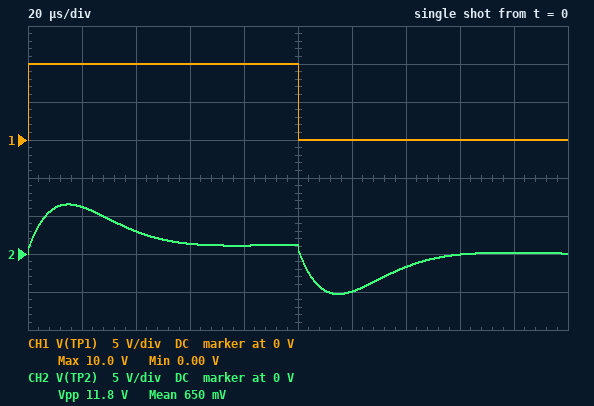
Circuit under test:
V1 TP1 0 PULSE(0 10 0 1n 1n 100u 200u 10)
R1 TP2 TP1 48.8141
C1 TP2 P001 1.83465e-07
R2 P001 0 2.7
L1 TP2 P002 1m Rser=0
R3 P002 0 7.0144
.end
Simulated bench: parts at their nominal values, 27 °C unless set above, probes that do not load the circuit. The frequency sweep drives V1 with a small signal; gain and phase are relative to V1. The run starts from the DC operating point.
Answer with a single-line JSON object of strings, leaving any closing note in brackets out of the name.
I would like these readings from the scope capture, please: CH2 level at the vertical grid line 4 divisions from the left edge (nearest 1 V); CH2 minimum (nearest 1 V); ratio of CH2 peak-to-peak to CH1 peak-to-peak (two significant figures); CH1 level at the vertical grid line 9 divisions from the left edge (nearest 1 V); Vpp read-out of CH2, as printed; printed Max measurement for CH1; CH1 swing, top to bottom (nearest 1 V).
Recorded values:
{"CH2 level at the vertical grid line 4 divisions from the left edge": "1 V", "CH2 minimum": "-5 V", "ratio of CH2 peak-to-peak to CH1 peak-to-peak": "1.2", "CH1 level at the vertical grid line 9 divisions from the left edge": "0 V", "Vpp read-out of CH2, as printed": "11.8 V", "printed Max measurement for CH1": "10.0 V", "CH1 swing, top to bottom": "10 V"}
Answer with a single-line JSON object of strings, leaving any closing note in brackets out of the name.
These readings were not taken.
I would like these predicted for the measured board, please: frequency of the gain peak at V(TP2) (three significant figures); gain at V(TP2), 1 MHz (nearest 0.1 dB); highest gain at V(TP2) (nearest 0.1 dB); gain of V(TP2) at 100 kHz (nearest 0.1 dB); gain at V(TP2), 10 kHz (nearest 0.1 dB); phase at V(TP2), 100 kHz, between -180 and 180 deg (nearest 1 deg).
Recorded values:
{"frequency of the gain peak at V(TP2)": "12.2 kHz", "gain at V(TP2), 1 MHz": "-25.2 dB", "highest gain at V(TP2)": "-0.7 dB", "gain of V(TP2) at 100 kHz": "-15.1 dB", "gain at V(TP2), 10 kHz": "-1.0 dB", "phase at V(TP2), 100 kHz, between -180 and 180 deg": "-63 deg"}
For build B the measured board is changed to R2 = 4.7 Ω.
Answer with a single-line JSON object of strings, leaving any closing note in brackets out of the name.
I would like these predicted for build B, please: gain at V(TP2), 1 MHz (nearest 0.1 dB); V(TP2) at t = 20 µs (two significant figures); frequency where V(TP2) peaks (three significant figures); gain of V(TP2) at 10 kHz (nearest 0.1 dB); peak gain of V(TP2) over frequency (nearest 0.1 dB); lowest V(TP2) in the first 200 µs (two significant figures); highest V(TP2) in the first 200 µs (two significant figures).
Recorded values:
{"gain at V(TP2), 1 MHz": "-21.0 dB", "V(TP2) at t = 20 µs": "6.1 V", "frequency where V(TP2) peaks": "12.0 kHz", "gain of V(TP2) at 10 kHz": "-1.1 dB", "peak gain of V(TP2) over frequency": "-0.9 dB", "lowest V(TP2) in the first 200 µs": "-5.2 V", "highest V(TP2) in the first 200 µs": "6.4 V"}
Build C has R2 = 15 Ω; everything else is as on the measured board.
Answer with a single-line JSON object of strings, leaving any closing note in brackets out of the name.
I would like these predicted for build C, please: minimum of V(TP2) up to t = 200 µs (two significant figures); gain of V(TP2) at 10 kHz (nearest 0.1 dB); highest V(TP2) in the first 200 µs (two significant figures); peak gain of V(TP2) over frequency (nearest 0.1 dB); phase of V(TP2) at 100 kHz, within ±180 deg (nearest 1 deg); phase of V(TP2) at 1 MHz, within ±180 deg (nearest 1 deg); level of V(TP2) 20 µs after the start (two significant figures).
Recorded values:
{"minimum of V(TP2) up to t = 200 µs": "-4.8 V", "gain of V(TP2) at 10 kHz": "-1.6 dB", "highest V(TP2) in the first 200 µs": "6.0 V", "peak gain of V(TP2) over frequency": "-1.5 dB", "phase of V(TP2) at 100 kHz, within ±180 deg": "-21 deg", "phase of V(TP2) at 1 MHz, within ±180 deg": "-2 deg", "level of V(TP2) 20 µs after the start": "5.7 V"}
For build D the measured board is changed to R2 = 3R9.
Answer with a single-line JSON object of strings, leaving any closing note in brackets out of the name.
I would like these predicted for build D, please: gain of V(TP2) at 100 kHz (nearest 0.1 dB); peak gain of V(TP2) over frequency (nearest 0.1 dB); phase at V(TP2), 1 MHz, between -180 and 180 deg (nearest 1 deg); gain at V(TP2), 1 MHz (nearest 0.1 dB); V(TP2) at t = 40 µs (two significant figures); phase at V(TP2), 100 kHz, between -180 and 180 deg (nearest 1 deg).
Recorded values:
{"gain of V(TP2) at 100 kHz": "-14.9 dB", "peak gain of V(TP2) over frequency": "-0.8 dB", "phase at V(TP2), 1 MHz, between -180 and 180 deg": "-12 deg", "gain at V(TP2), 1 MHz": "-22.4 dB", "V(TP2) at t = 40 µs": "3.0 V", "phase at V(TP2), 100 kHz, between -180 and 180 deg": "-56 deg"}
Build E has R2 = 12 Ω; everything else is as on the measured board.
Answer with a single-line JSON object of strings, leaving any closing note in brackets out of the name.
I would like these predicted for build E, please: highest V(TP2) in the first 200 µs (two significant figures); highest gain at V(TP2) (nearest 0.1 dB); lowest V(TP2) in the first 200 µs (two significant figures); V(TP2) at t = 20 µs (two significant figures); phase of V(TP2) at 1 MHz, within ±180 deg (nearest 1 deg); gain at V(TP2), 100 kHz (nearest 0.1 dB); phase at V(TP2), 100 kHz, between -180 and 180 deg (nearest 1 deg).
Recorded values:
{"highest V(TP2) in the first 200 µs": "6.1 V", "highest gain at V(TP2)": "-1.3 dB", "lowest V(TP2) in the first 200 µs": "-4.9 V", "V(TP2) at t = 20 µs": "5.8 V", "phase of V(TP2) at 1 MHz, within ±180 deg": "-3 deg", "gain at V(TP2), 100 kHz": "-12.3 dB", "phase at V(TP2), 100 kHz, between -180 and 180 deg": "-27 deg"}
